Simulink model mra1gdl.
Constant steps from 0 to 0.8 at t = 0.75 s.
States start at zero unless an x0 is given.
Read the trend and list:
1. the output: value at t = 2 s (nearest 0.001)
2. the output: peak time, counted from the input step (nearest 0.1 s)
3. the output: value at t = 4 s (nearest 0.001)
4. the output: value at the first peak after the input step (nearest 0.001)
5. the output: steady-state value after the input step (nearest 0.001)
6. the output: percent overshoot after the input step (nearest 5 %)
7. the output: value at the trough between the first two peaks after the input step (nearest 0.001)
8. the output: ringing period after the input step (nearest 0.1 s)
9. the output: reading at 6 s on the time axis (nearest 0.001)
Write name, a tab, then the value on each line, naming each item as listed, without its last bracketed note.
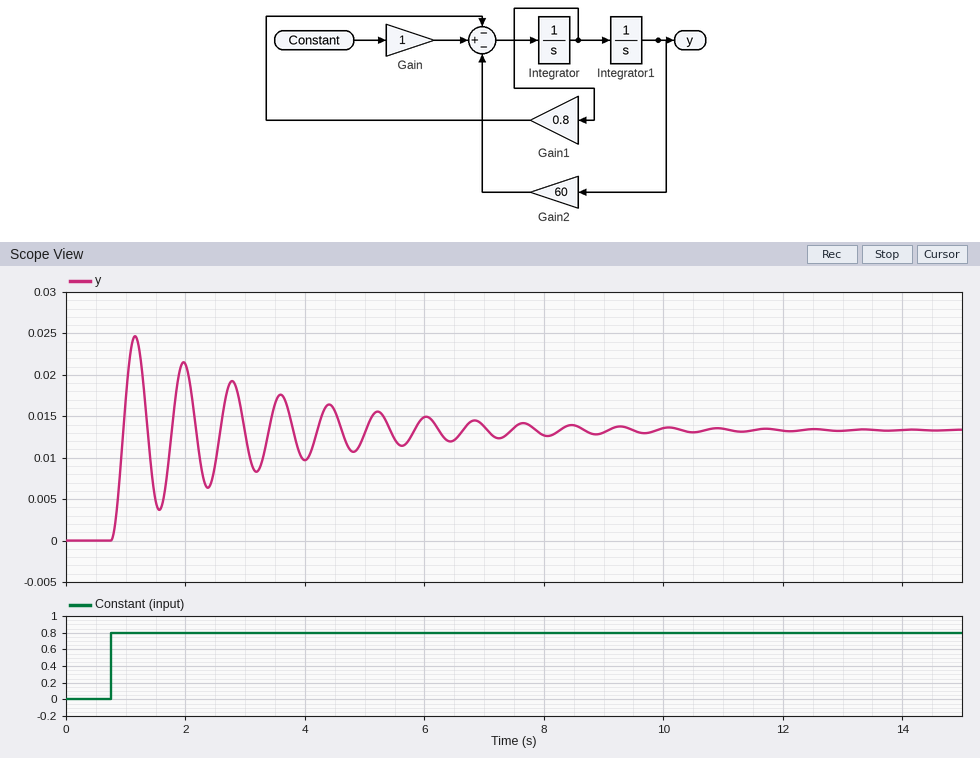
the output: value at t = 2 s	0.021
the output: peak time, counted from the input step	0.4 s
the output: value at t = 4 s	0.010
the output: value at the first peak after the input step	0.025
the output: steady-state value after the input step	0.013
the output: percent overshoot after the input step	85 %
the output: value at the trough between the first two peaks after the input step	0.004
the output: ringing period after the input step	0.8 s
the output: reading at 6 s on the time axis	0.015
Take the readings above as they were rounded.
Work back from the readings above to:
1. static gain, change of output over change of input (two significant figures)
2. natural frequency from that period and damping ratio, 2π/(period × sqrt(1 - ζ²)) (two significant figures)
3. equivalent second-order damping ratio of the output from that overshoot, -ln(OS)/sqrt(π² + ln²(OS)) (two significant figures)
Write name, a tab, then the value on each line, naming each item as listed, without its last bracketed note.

static gain, change of output over change of input	0.016
natural frequency from that period and damping ratio, 2π/(period × sqrt(1 - ζ²))	7.9 rad/s
equivalent second-order damping ratio of the output from that overshoot, -ln(OS)/sqrt(π² + ln²(OS))	0.052
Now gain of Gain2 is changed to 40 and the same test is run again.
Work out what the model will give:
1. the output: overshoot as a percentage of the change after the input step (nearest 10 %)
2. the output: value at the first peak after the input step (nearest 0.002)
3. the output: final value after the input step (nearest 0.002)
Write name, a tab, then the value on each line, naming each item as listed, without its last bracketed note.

the output: overshoot as a percentage of the change after the input step	80 %
the output: value at the first peak after the input step	0.036
the output: final value after the input step	0.020
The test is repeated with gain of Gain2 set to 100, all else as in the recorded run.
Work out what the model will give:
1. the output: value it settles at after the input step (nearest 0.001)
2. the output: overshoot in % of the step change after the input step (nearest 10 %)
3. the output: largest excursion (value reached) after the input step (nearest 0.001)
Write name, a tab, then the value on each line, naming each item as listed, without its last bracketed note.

the output: value it settles at after the input step	0.008
the output: overshoot in % of the step change after the input step	90 %
the output: largest excursion (value reached) after the input step	0.015
